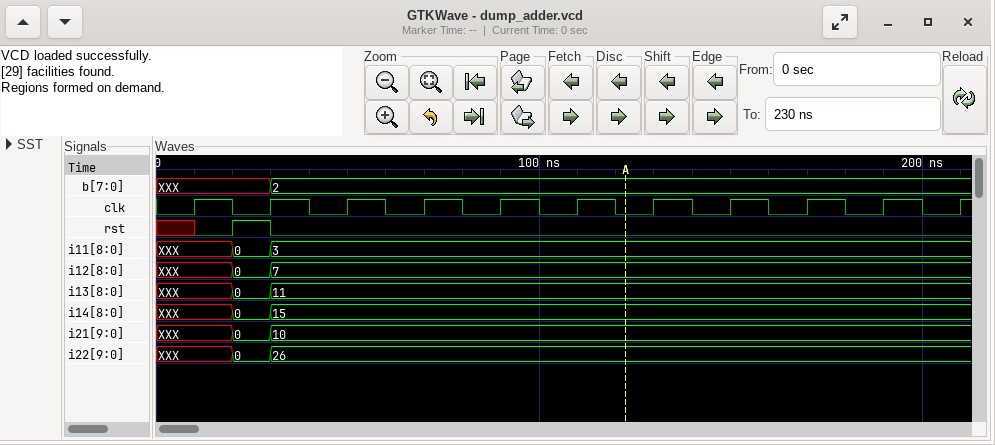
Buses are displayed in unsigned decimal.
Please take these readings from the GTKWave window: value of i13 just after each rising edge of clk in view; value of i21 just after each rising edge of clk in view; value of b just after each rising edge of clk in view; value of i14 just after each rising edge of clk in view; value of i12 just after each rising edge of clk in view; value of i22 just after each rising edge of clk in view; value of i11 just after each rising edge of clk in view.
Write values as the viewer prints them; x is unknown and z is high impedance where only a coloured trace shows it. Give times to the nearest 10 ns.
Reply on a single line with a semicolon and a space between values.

XXX, 11, 11, 11, 11, 11, 11, 11, 11, 11, 11; XXX, 10, 10, 10, 10, 10, 10, 10, 10, 10, 10; XXX, 2, 2, 2, 2, 2, 2, 2, 2, 2, 2; XXX, 15, 15, 15, 15, 15, 15, 15, 15, 15, 15; XXX, 7, 7, 7, 7, 7, 7, 7, 7, 7, 7; XXX, 26, 26, 26, 26, 26, 26, 26, 26, 26, 26; XXX, 3, 3, 3, 3, 3, 3, 3, 3, 3, 3
